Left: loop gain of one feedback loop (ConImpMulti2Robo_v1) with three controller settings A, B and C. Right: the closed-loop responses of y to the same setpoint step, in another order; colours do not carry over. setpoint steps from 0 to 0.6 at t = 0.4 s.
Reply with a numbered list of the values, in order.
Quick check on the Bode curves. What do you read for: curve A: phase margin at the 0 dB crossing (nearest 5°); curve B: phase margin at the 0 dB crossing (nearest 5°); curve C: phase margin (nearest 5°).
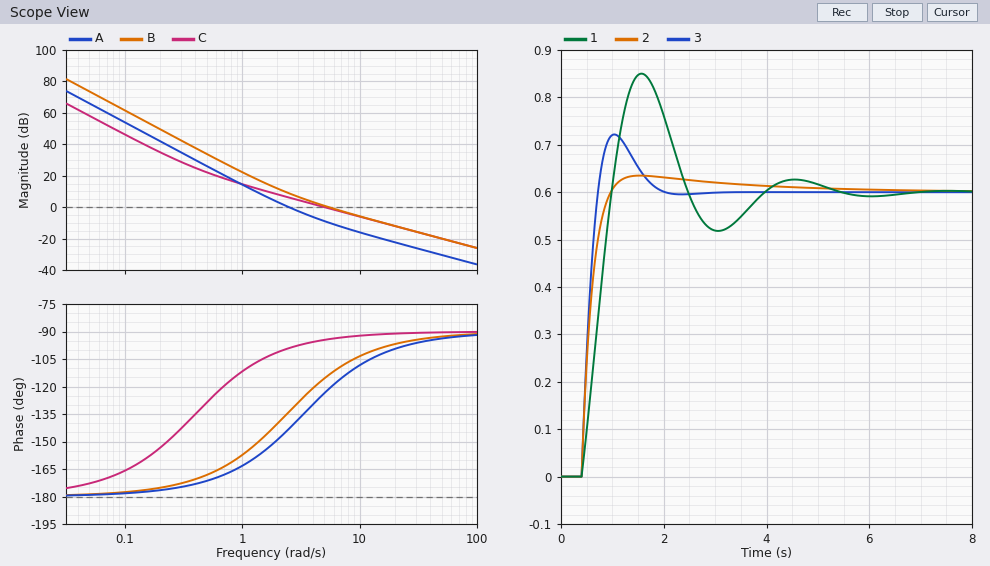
1. 35°
2. 65°
3. 85°
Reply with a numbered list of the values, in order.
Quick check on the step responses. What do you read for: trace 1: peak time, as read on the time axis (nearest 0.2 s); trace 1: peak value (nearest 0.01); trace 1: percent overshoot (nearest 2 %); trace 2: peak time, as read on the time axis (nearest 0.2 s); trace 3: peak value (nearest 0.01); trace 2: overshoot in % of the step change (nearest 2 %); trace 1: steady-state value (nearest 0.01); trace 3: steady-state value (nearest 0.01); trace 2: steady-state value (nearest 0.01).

1. 1.6 s
2. 0.85
3. 42 %
4. 1.6 s
5. 0.72
6. 6 %
7. 0.60
8. 0.60
9. 0.60
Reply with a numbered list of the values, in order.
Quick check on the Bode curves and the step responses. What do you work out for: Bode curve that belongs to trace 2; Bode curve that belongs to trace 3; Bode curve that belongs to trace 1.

1. C
2. B
3. A
